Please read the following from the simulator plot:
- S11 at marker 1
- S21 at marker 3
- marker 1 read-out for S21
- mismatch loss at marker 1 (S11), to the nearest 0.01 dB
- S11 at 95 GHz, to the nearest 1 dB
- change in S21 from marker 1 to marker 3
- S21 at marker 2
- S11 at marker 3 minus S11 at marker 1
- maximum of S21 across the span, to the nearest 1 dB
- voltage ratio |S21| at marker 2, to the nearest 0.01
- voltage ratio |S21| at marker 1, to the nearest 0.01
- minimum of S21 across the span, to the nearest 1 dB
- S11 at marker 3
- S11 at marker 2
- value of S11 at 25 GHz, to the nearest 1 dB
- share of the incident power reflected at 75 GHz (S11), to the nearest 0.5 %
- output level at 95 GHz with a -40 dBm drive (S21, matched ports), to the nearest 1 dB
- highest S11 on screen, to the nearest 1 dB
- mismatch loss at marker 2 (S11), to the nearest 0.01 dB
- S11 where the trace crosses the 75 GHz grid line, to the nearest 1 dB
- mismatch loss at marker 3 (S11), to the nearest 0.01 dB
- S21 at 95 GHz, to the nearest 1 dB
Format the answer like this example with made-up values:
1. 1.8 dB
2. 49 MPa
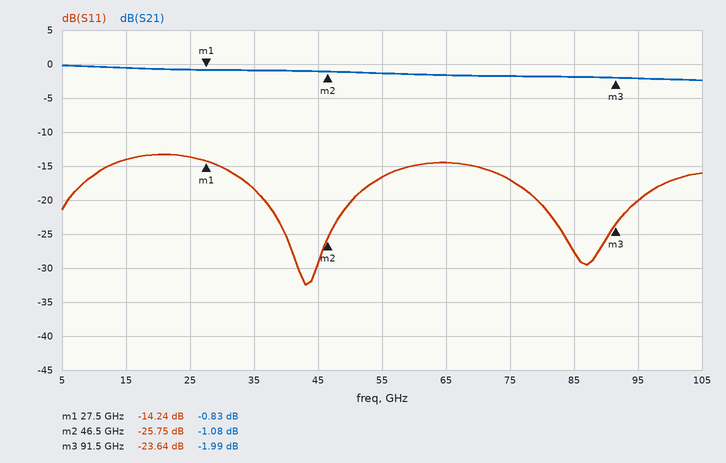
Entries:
1. -14.24 dB
2. -1.99 dB
3. -0.83 dB
4. 0.17 dB
5. -20 dB
6. -1.16 dB
7. -1.08 dB
8. -9.40 dB
9. 0 dB
10. 0.88
11. 0.91
12. -2 dB
13. -23.64 dB
14. -25.75 dB
15. -14 dB
16. 2.0 %
17. -42 dBm
18. -13 dB
19. 0.01 dB
20. -17 dB
21. 0.02 dB
22. -2 dB
